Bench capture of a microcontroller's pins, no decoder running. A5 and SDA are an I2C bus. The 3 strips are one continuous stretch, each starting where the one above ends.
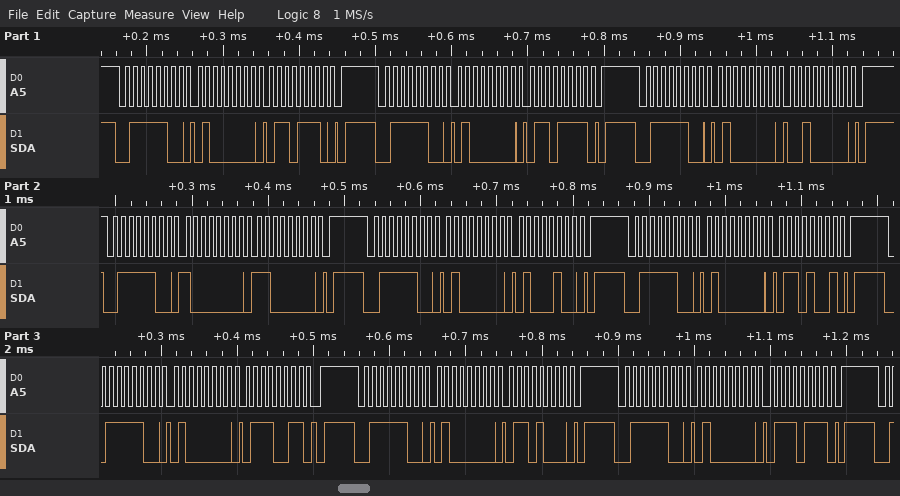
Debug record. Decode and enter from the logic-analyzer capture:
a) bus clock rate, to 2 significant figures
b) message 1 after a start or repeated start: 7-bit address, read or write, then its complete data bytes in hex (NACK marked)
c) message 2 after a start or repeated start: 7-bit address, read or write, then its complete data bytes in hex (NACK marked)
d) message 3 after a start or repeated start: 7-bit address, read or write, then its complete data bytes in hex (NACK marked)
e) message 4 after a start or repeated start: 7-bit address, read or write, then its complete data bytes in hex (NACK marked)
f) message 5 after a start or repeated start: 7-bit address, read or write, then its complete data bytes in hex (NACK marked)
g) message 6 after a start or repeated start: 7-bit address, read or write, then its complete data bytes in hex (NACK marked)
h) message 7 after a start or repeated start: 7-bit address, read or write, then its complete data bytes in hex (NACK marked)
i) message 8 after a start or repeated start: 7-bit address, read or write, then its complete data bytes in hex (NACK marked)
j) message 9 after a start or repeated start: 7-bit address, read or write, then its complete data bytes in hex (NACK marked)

100 kHz
0x3E write: 40 6E
0x3E write: 40 6F
0x3E write: 40 20
0x3E write: 80 C0
0x3E write: 40 44
0x3E write: 40 69
0x3E write: 40 73
0x3E write: 40 68
0x3E write: 40 77
